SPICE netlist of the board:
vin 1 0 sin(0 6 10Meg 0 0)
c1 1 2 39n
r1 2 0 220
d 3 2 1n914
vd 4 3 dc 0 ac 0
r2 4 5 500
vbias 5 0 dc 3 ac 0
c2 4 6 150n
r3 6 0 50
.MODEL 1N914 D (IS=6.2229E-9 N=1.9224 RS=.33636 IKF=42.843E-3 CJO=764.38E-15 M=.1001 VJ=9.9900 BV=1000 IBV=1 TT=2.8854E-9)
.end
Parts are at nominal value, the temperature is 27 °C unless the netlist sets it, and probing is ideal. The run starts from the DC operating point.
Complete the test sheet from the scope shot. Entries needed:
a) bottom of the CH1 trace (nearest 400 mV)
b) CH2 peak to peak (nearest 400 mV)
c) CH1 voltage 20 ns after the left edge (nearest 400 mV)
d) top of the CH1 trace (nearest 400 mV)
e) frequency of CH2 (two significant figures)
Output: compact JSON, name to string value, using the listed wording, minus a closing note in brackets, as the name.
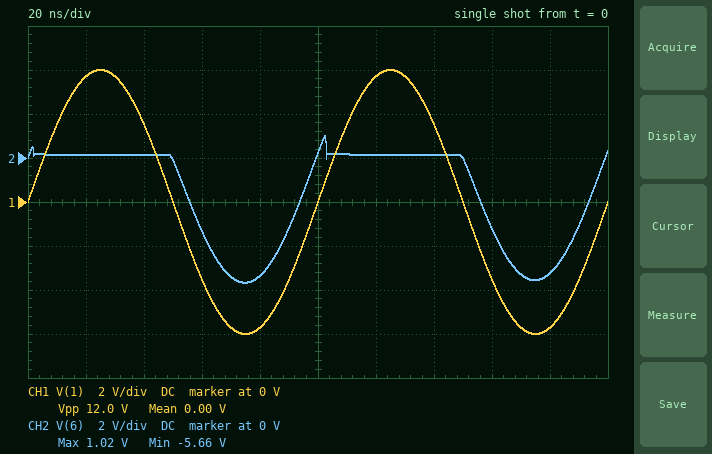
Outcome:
{"bottom of the CH1 trace": "-6.0 V", "CH2 peak to peak": "6.8 V", "CH1 voltage 20 ns after the left edge": "5.6 V", "top of the CH1 trace": "6.0 V", "frequency of CH2": "10 MHz"}
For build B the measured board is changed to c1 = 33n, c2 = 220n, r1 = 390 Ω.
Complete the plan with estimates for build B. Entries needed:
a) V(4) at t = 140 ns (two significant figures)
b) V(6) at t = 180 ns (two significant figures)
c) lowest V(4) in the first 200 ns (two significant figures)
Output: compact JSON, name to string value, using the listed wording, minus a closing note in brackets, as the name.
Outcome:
{"V(4) at t = 140 ns": "1.8 V", "V(6) at t = 180 ns": "-5.2 V", "lowest V(4) in the first 200 ns": "-4.0 V"}
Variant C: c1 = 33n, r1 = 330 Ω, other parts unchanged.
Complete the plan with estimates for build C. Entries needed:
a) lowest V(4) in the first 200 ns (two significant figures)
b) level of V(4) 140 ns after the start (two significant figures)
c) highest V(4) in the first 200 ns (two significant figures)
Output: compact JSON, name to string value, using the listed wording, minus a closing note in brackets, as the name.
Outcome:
{"lowest V(4) in the first 200 ns": "-4.1 V", "level of V(4) 140 ns after the start": "1.7 V", "highest V(4) in the first 200 ns": "2.6 V"}
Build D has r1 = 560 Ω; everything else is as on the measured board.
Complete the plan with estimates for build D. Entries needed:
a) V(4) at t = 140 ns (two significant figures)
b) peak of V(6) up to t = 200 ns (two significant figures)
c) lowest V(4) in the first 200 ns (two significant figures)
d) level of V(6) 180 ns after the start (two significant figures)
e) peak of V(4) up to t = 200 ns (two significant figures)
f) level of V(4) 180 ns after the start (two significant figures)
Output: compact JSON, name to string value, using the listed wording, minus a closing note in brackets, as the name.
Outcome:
{"V(4) at t = 140 ns": "2.0 V", "peak of V(6) up to t = 200 ns": "970 mV", "lowest V(4) in the first 200 ns": "-3.8 V", "level of V(6) 180 ns after the start": "-5.2 V", "peak of V(4) up to t = 200 ns": "2.8 V", "level of V(4) 180 ns after the start": "-3.4 V"}
